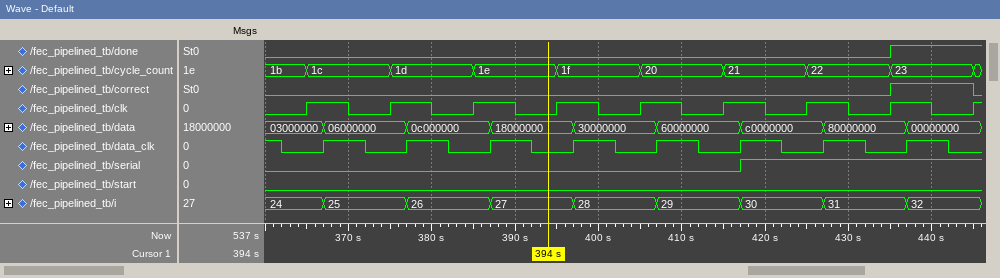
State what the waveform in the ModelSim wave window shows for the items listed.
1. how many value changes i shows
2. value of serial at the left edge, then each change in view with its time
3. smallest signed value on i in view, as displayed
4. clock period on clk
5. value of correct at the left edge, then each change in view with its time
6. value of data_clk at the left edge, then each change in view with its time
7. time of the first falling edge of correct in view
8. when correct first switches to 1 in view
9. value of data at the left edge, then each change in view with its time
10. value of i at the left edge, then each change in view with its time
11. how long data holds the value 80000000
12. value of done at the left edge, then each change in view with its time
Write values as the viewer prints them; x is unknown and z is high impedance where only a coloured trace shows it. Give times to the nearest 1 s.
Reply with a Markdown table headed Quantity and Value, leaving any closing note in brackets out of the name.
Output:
| Quantity | Value |
|---|---|
| how many value changes i shows | 8 |
| value of serial at the left edge, then each change in view with its time | 0, 1 at 417 s |
| smallest signed value on i in view, as displayed | 24 |
| clock period on clk | 10 s |
| value of correct at the left edge, then each change in view with its time | 0, 1 at 435 s, 0 at 445 s |
| value of data_clk at the left edge, then each change in view with its time | 1, 0 at 362 s, 1 at 367 s, 0 at 372 s, 1 at 377 s, 0 at 382 s, 1 at 387 s, 0 at 392 s, 1 at 397 s, 0 at 402 s, 1 at 407 s, 0 at 412 s, 1 at 417 s, 0 at 422 s, 1 at 427 s, 0 at 432 s, 1 at 437 s, 0 at 442 s |
| time of the first falling edge of correct in view | 445 s |
| when correct first switches to 1 in view | 435 s |
| value of data at the left edge, then each change in view with its time | 03000000, 06000000 at 367 s, 0c000000 at 377 s, 18000000 at 387 s, 30000000 at 397 s, 60000000 at 407 s, c0000000 at 417 s, 80000000 at 427 s, 00000000 at 437 s |
| value of i at the left edge, then each change in view with its time | 24, 25 at 367 s, 26 at 377 s, 27 at 387 s, 28 at 397 s, 29 at 407 s, 30 at 417 s, 31 at 427 s, 32 at 437 s |
| how long data holds the value 80000000 | 10 s |
| value of done at the left edge, then each change in view with its time | 0, 1 at 435 s |
